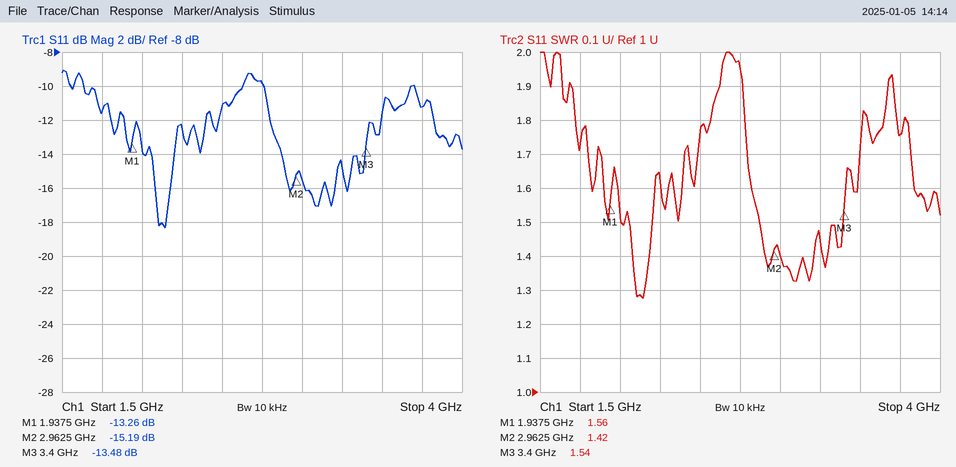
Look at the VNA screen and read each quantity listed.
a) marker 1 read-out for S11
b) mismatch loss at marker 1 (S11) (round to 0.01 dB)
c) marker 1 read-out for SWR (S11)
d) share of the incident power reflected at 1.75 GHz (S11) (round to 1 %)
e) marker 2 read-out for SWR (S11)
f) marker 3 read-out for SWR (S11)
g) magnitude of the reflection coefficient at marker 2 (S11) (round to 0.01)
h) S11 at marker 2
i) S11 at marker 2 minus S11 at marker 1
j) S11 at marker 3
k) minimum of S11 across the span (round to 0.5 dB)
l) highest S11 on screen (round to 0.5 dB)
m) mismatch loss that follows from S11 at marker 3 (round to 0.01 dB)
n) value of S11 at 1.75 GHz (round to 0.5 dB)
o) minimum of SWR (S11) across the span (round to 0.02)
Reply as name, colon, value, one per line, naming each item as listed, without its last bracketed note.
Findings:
marker 1 read-out for S11: -13.26 dB
mismatch loss at marker 1 (S11): 0.21 dB
marker 1 read-out for SWR: 1.56
share of the incident power reflected at 1.75 GHz (S11): 7 %
marker 2 read-out for SWR: 1.42
marker 3 read-out for SWR: 1.54
magnitude of the reflection coefficient at marker 2 (S11): 0.17
S11 at marker 2: -15.19 dB
S11 at marker 2 minus S11 at marker 1: -1.93 dB
S11 at marker 3: -13.48 dB
minimum of S11 across the span: -18.5 dB
highest S11 on screen: -9.0 dB
mismatch loss that follows from S11 at marker 3: 0.20 dB
value of S11 at 1.75 GHz: -11.5 dB
minimum of SWR (S11) across the span: 1.28
